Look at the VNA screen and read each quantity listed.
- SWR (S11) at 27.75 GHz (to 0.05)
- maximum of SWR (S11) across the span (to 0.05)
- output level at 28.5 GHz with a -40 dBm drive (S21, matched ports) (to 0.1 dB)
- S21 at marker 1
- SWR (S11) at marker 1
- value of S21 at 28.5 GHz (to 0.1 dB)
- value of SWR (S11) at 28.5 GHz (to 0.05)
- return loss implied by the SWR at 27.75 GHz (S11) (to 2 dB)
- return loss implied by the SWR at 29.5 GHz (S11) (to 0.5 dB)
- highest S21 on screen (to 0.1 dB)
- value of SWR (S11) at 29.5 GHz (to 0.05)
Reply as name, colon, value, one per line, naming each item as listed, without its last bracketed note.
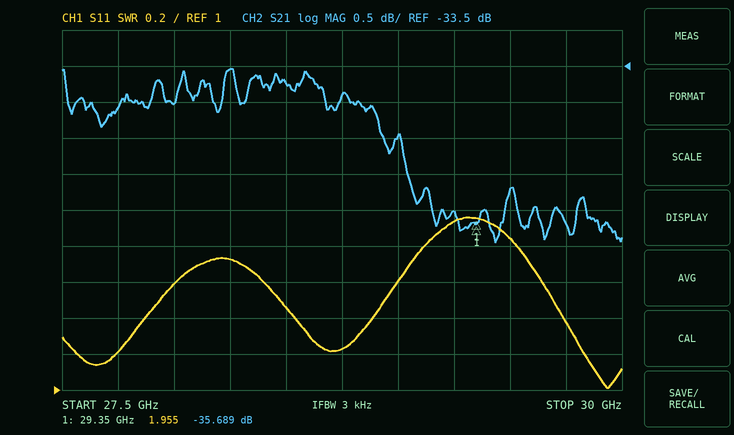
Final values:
SWR (S11) at 27.75 GHz: 1.20
maximum of SWR (S11) across the span: 1.95
output level at 28.5 GHz with a -40 dBm drive (S21, matched ports): -73.7 dBm
S21 at marker 1: -35.689 dB
SWR (S11) at marker 1: 1.955
value of S21 at 28.5 GHz: -33.7 dB
value of SWR (S11) at 28.5 GHz: 1.45
return loss implied by the SWR at 27.75 GHz (S11): 20 dB
return loss implied by the SWR at 29.5 GHz (S11): 10.5 dB
highest S21 on screen: -33.5 dB
value of SWR (S11) at 29.5 GHz: 1.85
